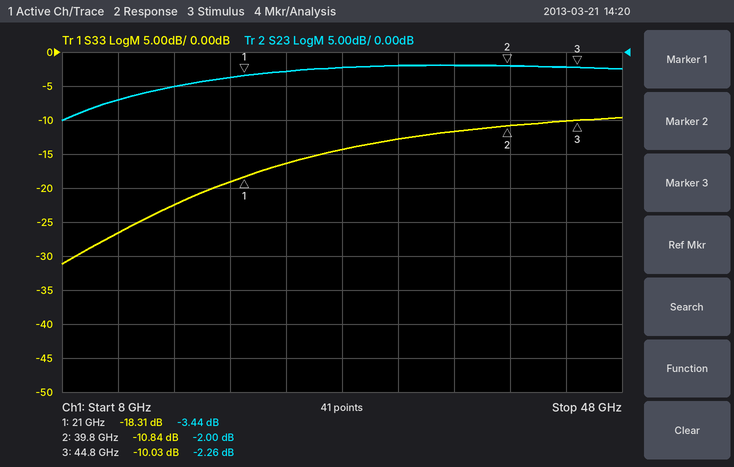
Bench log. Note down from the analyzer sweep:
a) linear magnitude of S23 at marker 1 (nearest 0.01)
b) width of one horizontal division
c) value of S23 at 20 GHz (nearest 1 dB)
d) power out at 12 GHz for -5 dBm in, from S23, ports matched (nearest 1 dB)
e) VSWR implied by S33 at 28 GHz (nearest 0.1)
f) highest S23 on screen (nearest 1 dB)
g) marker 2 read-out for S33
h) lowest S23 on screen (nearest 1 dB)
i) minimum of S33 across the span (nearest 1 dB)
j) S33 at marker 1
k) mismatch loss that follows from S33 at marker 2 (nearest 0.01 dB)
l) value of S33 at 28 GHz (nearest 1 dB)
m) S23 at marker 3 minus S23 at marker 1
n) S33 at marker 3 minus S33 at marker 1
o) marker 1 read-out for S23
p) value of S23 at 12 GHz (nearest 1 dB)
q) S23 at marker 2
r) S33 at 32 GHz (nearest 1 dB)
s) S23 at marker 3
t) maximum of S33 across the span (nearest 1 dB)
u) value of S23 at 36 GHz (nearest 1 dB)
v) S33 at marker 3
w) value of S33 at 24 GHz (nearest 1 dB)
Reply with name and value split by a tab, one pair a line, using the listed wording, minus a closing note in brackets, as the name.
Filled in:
linear magnitude of S23 at marker 1	0.67
width of one horizontal division	4 GHz
value of S23 at 20 GHz	-4 dB
power out at 12 GHz for -5 dBm in, from S23, ports matched	-12 dBm
VSWR implied by S33 at 28 GHz	1.5
highest S23 on screen	-2 dB
marker 2 read-out for S33	-10.84 dB
lowest S23 on screen	-10 dB
minimum of S33 across the span	-31 dB
S33 at marker 1	-18.31 dB
mismatch loss that follows from S33 at marker 2	0.37 dB
value of S33 at 28 GHz	-14 dB
S23 at marker 3 minus S23 at marker 1	1.18 dB
S33 at marker 3 minus S33 at marker 1	8.28 dB
marker 1 read-out for S23	-3.44 dB
value of S23 at 12 GHz	-7 dB
S23 at marker 2	-2.00 dB
S33 at 32 GHz	-13 dB
S23 at marker 3	-2.26 dB
maximum of S33 across the span	-10 dB
value of S23 at 36 GHz	-2 dB
S33 at marker 3	-10.03 dB
value of S33 at 24 GHz	-16 dB
